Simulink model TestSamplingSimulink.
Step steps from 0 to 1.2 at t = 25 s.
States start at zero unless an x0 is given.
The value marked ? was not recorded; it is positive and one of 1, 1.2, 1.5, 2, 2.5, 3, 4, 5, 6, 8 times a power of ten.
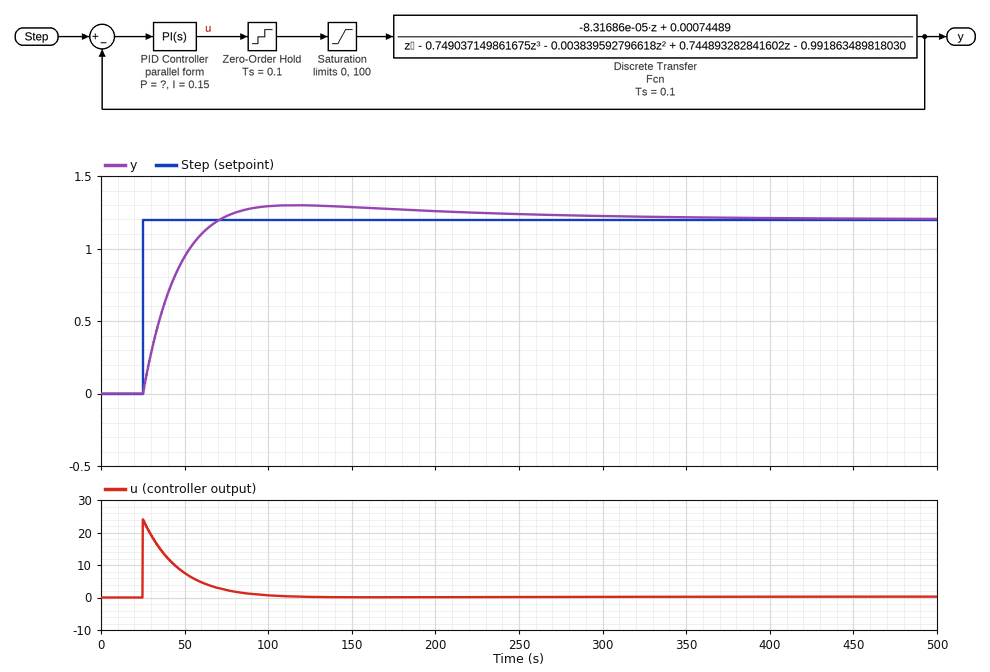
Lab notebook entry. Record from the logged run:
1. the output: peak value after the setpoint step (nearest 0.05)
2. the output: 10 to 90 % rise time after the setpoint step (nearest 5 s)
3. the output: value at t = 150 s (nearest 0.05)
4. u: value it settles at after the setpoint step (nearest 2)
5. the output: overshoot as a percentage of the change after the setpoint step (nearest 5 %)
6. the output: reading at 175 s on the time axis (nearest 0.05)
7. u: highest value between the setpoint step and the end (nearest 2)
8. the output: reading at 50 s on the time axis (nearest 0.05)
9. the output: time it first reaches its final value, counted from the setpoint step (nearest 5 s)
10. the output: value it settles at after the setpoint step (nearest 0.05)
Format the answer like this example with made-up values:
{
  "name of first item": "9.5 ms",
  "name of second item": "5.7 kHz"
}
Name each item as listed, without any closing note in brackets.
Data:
{
  "the output: peak value after the setpoint step": "1.30",
  "the output: 10 to 90 % rise time after the setpoint step": "30 s",
  "the output: value at t = 150 s": "1.30",
  "u: value it settles at after the setpoint step": "0",
  "the output: overshoot as a percentage of the change after the setpoint step": "10 %",
  "the output: reading at 175 s on the time axis": "1.25",
  "u: highest value between the setpoint step and the end": "24",
  "the output: reading at 50 s on the time axis": "0.95",
  "the output: time it first reaches its final value, counted from the setpoint step": "45 s",
  "the output: value it settles at after the setpoint step": "1.20"
}
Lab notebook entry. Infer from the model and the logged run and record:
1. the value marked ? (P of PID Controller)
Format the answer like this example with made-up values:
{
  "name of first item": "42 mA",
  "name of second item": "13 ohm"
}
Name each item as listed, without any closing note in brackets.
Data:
{
  "the value marked ?": "20"
}
